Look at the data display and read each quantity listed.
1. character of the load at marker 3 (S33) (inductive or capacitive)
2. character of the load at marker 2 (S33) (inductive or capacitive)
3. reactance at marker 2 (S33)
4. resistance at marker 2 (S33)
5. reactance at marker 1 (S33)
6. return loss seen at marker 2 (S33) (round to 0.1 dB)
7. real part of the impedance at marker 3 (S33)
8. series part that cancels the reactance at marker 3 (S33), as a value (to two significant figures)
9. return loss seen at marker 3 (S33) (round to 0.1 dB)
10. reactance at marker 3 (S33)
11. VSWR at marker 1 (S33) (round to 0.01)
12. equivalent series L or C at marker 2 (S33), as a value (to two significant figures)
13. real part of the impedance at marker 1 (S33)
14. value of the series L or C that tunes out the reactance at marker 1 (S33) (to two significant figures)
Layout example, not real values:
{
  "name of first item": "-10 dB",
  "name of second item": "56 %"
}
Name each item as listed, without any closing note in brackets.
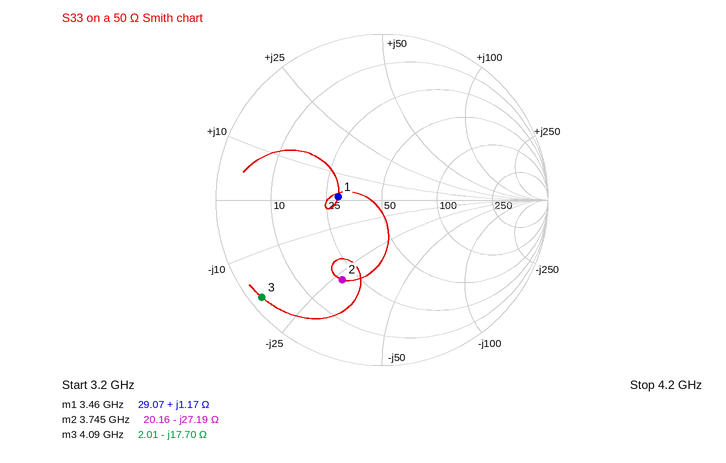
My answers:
{
  "character of the load at marker 3 (S33)": "capacitive",
  "character of the load at marker 2 (S33)": "capacitive",
  "reactance at marker 2": "-27.19 Ω",
  "resistance at marker 2": "20.16 Ω",
  "reactance at marker 1": "+1.17 Ω",
  "return loss seen at marker 2 (S33)": "5.4 dB",
  "real part of the impedance at marker 3": "2.01 Ω",
  "series part that cancels the reactance at marker 3 (S33), as a value": "690 pH",
  "return loss seen at marker 3 (S33)": "0.6 dB",
  "reactance at marker 3": "-17.70 Ω",
  "VSWR at marker 1 (S33)": "1.72",
  "equivalent series L or C at marker 2 (S33), as a value": "1.6 pF",
  "real part of the impedance at marker 1": "29.07 Ω",
  "value of the series L or C that tunes out the reactance at marker 1 (S33)": "39 pF"
}
